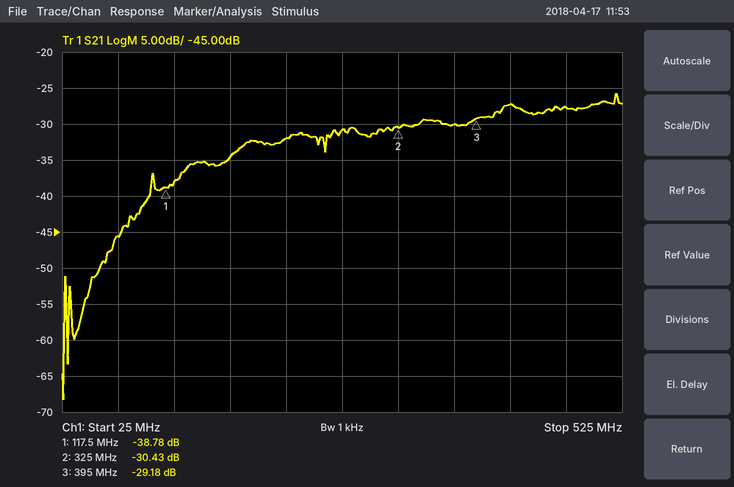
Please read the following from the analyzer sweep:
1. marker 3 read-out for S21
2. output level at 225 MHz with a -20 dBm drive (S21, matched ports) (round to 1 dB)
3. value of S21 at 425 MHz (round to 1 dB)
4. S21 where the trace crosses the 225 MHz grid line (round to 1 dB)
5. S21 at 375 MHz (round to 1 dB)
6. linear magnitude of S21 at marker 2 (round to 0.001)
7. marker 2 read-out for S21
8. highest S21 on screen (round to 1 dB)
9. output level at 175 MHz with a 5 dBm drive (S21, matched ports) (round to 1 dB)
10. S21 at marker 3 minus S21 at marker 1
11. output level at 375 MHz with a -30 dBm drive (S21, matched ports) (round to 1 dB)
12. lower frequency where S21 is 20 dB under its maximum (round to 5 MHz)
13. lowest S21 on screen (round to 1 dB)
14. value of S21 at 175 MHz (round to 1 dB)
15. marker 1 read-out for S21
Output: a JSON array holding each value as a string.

["-29.18 dB", "-52 dBm", "-27 dB", "-32 dB", "-30 dB", "0.030", "-30.43 dB", "-26 dB", "-30 dBm", "9.60 dB", "-60 dBm", "75 MHz", "-68 dB", "-35 dB", "-38.78 dB"]
